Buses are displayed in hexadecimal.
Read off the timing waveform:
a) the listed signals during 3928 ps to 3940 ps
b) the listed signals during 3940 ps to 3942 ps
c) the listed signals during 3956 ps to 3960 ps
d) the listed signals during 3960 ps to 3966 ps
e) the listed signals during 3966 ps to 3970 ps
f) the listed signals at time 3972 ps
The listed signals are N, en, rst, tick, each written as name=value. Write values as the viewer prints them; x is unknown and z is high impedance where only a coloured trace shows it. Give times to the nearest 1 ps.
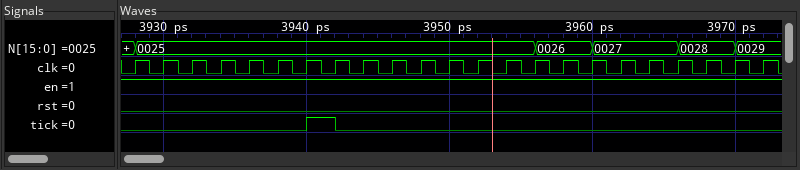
N=0025, en=1, rst=0, tick=0
N=0025, en=1, rst=0, tick=1
N=0026, en=1, rst=0, tick=0
N=0027, en=1, rst=0, tick=0
N=0028, en=1, rst=0, tick=0
N=0029, en=1, rst=0, tick=0
